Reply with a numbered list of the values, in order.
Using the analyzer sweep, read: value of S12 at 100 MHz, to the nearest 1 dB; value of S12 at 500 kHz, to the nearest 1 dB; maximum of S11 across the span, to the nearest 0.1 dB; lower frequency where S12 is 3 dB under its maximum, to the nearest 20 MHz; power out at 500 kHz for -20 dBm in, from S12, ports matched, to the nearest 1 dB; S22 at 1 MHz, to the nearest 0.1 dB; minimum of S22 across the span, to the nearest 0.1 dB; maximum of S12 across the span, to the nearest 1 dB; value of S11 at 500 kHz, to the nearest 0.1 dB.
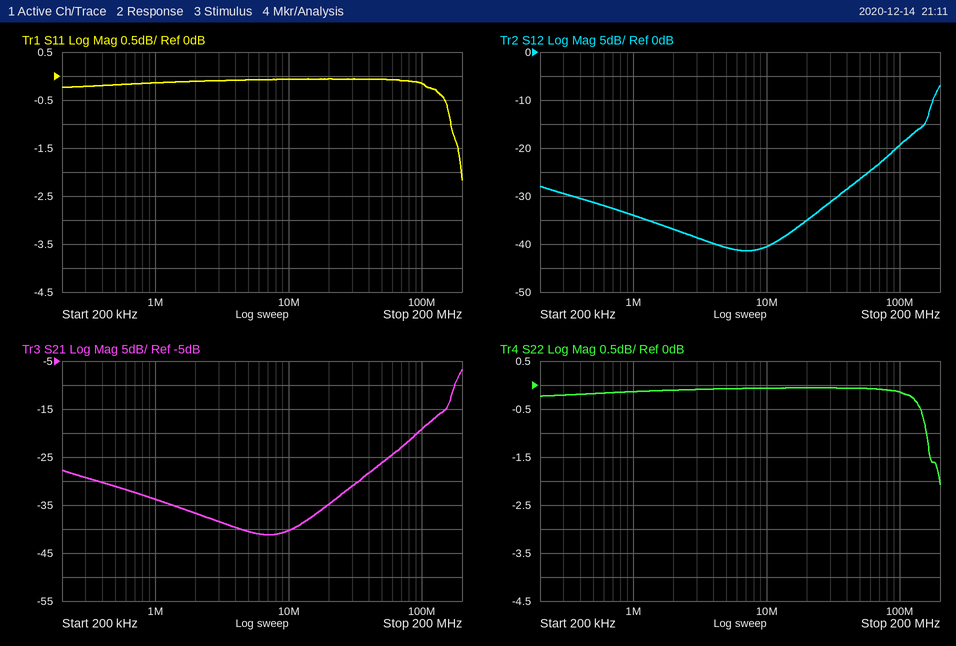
1. -19 dB
2. -31 dB
3. -0.1 dB
4. 180 MHz
5. -51 dBm
6. -0.1 dB
7. -2.1 dB
8. -7 dB
9. -0.2 dB
